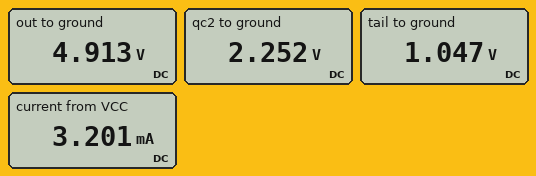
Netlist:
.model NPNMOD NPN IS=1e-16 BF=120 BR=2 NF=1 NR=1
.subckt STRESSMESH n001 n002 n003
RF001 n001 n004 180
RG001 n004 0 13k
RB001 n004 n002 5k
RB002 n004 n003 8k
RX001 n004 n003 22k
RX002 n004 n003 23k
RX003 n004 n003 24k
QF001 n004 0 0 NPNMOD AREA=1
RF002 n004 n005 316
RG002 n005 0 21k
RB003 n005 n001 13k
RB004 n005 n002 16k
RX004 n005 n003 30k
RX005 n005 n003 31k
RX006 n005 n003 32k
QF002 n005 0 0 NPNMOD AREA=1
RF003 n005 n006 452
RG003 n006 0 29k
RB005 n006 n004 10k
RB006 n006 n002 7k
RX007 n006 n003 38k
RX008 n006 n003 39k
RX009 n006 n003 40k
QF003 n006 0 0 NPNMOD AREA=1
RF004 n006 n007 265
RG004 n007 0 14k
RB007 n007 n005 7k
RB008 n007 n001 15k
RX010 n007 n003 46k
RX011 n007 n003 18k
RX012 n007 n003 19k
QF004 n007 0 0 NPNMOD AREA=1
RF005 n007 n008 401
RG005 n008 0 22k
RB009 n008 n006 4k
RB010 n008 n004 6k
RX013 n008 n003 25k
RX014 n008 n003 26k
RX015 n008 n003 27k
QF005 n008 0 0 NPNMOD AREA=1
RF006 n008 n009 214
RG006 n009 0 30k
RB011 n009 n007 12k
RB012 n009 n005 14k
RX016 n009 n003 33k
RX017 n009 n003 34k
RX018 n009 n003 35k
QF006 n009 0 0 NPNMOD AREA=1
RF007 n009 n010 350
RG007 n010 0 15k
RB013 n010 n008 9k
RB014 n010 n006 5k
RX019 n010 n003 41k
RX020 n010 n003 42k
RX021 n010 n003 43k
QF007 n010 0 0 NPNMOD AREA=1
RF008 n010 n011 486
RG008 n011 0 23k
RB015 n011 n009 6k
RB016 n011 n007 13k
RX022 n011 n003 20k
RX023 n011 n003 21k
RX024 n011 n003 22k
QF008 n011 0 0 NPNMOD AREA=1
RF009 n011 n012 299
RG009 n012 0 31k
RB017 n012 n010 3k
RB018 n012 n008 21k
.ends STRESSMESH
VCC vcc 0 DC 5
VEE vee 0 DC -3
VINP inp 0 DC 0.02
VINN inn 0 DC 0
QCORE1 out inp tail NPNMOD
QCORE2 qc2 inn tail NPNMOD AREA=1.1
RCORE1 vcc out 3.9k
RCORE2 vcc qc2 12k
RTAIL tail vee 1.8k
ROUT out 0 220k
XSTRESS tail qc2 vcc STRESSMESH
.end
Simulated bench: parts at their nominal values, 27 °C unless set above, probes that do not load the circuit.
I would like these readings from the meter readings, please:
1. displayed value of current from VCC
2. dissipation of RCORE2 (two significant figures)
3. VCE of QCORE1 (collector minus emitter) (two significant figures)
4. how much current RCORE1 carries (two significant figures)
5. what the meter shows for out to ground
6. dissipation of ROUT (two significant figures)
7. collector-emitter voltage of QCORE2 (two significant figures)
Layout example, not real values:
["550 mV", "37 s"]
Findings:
["3.201 mA", "630 µW", "3.9 V", "22 µA", "4.913 V", "110 µW", "1.2 V"]
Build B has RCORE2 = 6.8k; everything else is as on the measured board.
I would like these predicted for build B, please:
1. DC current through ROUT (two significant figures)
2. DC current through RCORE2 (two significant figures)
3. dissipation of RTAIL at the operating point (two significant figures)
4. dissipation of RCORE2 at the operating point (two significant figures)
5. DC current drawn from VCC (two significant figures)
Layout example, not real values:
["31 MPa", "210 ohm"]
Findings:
["22 µA", "350 µA", "9.4 mW", "830 µW", "3.3 mA"]
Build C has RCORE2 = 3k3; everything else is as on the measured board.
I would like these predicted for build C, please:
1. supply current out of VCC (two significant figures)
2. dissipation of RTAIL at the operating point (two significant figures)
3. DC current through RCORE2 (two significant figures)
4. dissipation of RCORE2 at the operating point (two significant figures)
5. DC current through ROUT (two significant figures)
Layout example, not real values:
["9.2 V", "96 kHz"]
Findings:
["3.4 mA", "9.9 mW", "540 µA", "970 µW", "22 µA"]
